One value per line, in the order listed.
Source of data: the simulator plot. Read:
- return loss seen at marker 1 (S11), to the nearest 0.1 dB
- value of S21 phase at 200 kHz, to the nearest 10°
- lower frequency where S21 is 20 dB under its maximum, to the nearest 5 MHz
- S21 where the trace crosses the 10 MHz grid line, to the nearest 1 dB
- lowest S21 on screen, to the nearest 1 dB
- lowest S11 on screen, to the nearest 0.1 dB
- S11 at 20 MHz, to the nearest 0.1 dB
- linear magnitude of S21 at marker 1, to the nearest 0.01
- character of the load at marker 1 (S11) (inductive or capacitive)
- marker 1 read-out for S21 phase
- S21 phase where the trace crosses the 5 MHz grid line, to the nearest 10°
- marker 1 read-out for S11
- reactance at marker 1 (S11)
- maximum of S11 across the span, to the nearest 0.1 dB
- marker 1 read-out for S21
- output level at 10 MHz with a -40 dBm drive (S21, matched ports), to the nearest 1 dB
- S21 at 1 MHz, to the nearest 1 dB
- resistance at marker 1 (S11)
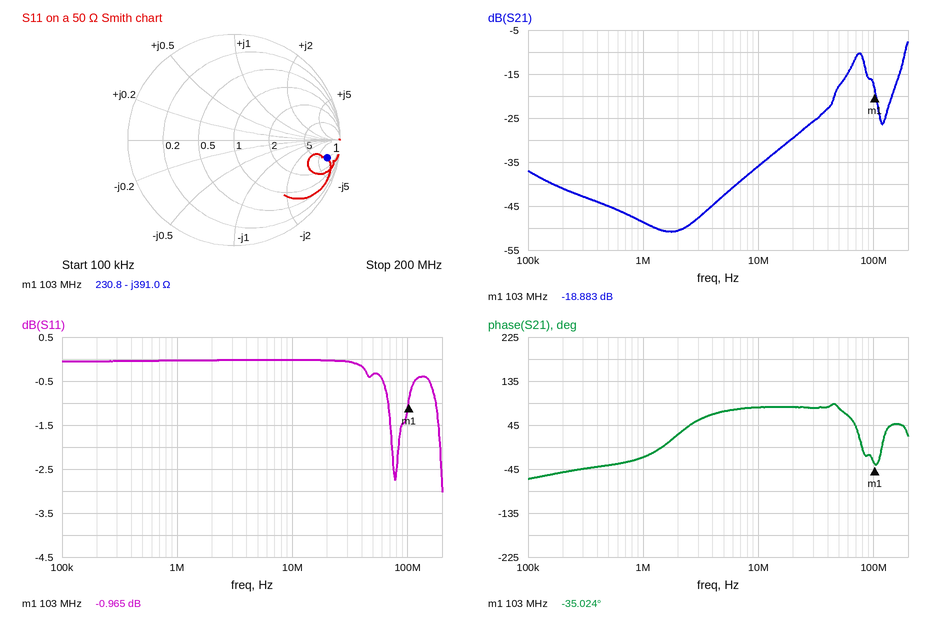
1.0 dB
-50°
25 MHz
-36 dB
-51 dB
-3.0 dB
0.0 dB
0.11
capacitive
-35.024°
70°
-0.965 dB
-391.0 Ω
0.0 dB
-18.883 dB
-76 dBm
-49 dB
230.8 Ω
